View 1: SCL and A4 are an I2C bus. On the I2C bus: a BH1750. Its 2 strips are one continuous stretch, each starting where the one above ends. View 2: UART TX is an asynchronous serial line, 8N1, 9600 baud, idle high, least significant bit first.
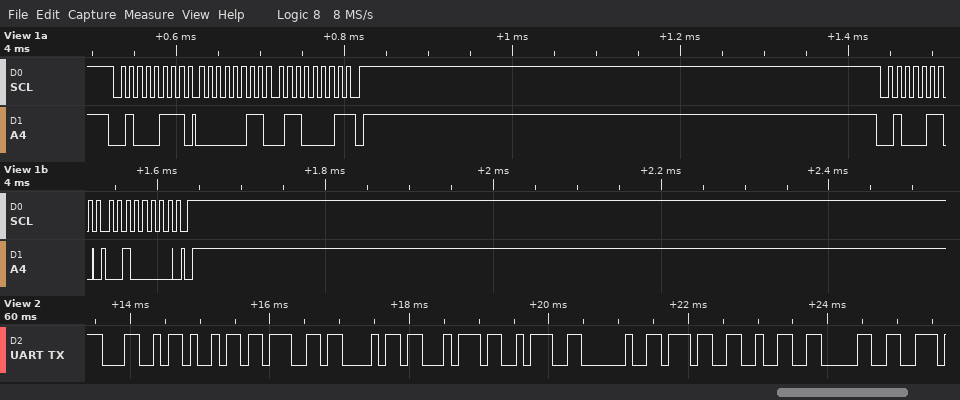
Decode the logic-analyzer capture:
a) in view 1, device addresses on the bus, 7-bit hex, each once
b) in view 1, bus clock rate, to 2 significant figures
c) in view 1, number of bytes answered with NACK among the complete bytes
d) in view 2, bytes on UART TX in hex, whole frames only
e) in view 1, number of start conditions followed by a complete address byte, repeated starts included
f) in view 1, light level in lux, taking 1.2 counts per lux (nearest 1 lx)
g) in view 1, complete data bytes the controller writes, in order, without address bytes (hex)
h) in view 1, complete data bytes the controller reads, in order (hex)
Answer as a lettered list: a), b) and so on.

a) 0x23
b) 100 kHz
c) 1
d) 0x4C 0x69 0x67 0x68 0x74 0x3A 0x20 0x37 0x32 0x30
e) 2
f) 721 lx
g) 20
h) 03 61
